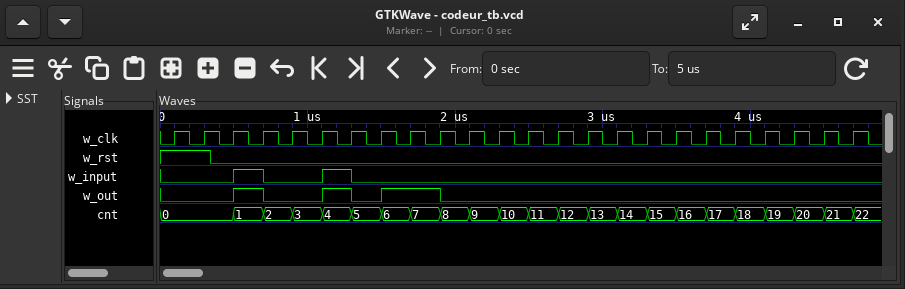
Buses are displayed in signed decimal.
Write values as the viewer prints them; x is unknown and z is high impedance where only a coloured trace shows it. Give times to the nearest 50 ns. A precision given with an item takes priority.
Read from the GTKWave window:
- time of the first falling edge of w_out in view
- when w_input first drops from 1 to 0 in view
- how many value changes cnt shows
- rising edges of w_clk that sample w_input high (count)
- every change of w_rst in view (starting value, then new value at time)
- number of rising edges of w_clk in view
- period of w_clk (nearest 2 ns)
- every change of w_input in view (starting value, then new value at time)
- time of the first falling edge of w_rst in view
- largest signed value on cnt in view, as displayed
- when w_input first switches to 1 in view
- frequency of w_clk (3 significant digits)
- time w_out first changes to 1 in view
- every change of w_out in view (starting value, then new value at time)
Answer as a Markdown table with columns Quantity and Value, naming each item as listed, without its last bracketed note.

| Quantity | Value |
|---|---|
| time of the first falling edge of w_out in view | 700 ns |
| when w_input first drops from 1 to 0 in view | 700 ns |
| how many value changes cnt shows | 22 |
| rising edges of w_clk that sample w_input high | 2 |
| every change of w_rst in view | 1, 0 at 350 ns |
| number of rising edges of w_clk in view | 24 |
| period of w_clk | 200 ns |
| every change of w_input in view | 0, 1 at 500 ns, 0 at 700 ns, 1 at 1100 ns, 0 at 1300 ns |
| time of the first falling edge of w_rst in view | 350 ns |
| largest signed value on cnt in view, as displayed | 22 |
| when w_input first switches to 1 in view | 500 ns |
| frequency of w_clk | 5.00 MHz |
| time w_out first changes to 1 in view | 500 ns |
| every change of w_out in view | 0, 1 at 500 ns, 0 at 700 ns, 1 at 1100 ns, 0 at 1300 ns, 1 at 1500 ns, 0 at 1900 ns |
